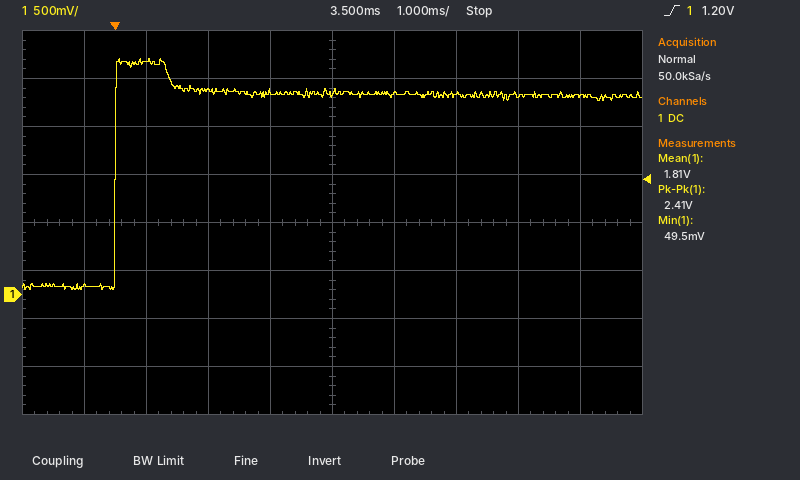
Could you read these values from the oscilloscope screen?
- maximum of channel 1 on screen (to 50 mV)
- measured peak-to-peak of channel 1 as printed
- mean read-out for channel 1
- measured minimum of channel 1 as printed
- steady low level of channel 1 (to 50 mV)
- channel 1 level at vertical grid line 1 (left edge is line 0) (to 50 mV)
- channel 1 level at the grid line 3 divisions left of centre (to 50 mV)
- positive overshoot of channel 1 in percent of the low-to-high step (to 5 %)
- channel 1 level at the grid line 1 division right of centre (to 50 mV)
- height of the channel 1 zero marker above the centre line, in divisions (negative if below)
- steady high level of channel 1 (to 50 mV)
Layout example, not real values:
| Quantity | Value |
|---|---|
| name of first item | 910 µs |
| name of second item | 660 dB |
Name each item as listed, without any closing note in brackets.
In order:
| Quantity | Value |
|---|---|
| maximum of channel 1 on screen | 2.45 V |
| measured peak-to-peak of channel 1 as printed | 2.41 V |
| mean read-out for channel 1 | 1.81 V |
| measured minimum of channel 1 as printed | 49.5 mV |
| steady low level of channel 1 | 100 mV |
| channel 1 level at vertical grid line 1 (left edge is line 0) | 100 mV |
| channel 1 level at the grid line 3 divisions left of centre | 2.45 V |
| positive overshoot of channel 1 in percent of the low-to-high step | 20 % |
| channel 1 level at the grid line 1 division right of centre | 2.10 V |
| height of the channel 1 zero marker above the centre line, in divisions | -1.5 div |
| steady high level of channel 1 | 2.10 V |
